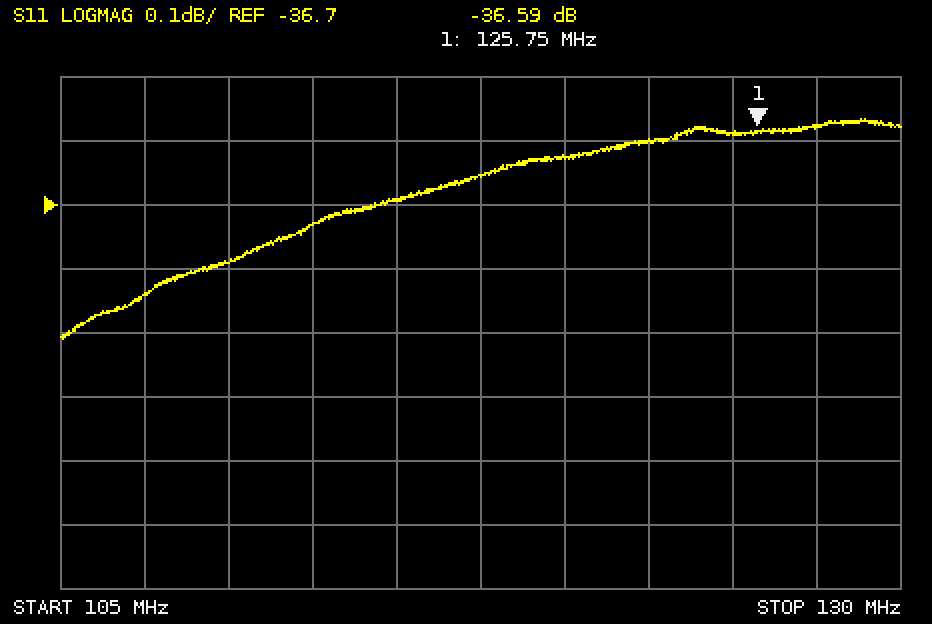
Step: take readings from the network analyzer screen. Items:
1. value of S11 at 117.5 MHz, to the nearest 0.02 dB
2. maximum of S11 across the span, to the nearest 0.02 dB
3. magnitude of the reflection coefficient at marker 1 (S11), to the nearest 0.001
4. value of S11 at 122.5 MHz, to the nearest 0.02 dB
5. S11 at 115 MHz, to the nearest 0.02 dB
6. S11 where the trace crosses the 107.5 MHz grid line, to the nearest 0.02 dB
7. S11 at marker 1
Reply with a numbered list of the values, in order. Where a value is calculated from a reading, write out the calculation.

1. -36.66 dB
2. -36.56 dB
3. 10^(-36.59/20) ≈ 0.015
4. -36.60 dB
5. -36.70 dB
6. -36.84 dB
7. -36.59 dB
